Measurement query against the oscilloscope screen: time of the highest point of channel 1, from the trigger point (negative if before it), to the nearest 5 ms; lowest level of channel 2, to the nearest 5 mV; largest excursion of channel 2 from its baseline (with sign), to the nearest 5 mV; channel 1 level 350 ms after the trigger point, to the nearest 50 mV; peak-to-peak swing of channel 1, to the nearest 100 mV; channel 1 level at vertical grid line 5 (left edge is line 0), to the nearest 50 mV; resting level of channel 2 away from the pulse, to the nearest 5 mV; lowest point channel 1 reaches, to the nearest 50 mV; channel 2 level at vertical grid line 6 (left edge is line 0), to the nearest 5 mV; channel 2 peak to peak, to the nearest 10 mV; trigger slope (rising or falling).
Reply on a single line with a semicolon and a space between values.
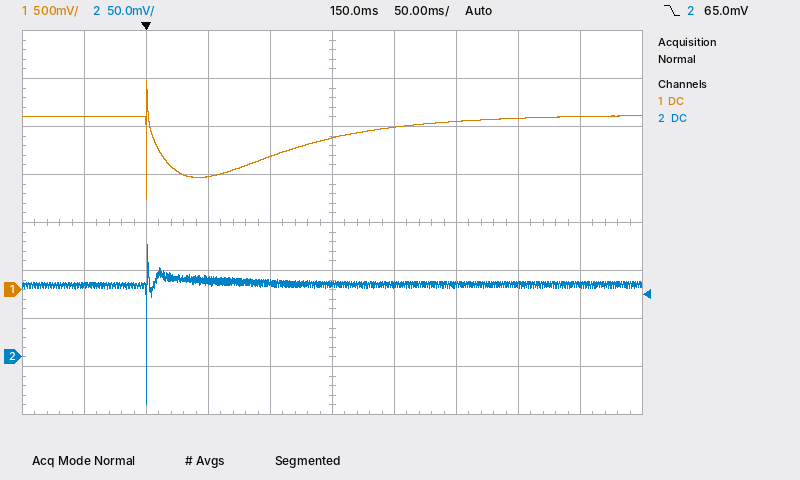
0 ms; -50 mV; -125 mV; 1.80 V; 1.20 V; 1.60 V; 75 mV; 950 mV; 75 mV; 170 mV; falling
